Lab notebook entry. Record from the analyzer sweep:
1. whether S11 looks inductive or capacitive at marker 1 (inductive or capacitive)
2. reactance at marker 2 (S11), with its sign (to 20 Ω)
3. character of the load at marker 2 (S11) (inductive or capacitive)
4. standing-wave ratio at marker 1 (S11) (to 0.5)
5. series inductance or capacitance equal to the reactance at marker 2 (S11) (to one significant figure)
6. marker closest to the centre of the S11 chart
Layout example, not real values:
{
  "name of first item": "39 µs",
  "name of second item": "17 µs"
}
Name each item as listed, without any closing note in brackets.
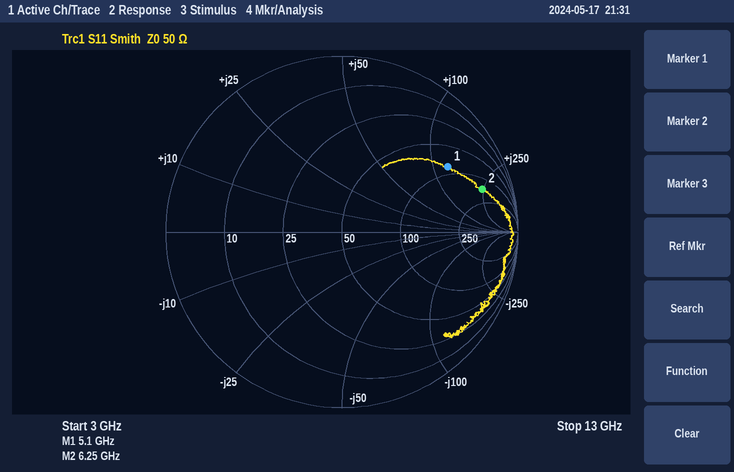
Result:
{
  "whether S11 looks inductive or capacitive at marker 1": "inductive",
  "reactance at marker 2 (S11), with its sign": "+240 Ω",
  "character of the load at marker 2 (S11)": "inductive",
  "standing-wave ratio at marker 1 (S11)": "6.0",
  "series inductance or capacitance equal to the reactance at marker 2 (S11)": "6 nH",
  "marker closest to the centre of the S11 chart": "marker 1"
}
